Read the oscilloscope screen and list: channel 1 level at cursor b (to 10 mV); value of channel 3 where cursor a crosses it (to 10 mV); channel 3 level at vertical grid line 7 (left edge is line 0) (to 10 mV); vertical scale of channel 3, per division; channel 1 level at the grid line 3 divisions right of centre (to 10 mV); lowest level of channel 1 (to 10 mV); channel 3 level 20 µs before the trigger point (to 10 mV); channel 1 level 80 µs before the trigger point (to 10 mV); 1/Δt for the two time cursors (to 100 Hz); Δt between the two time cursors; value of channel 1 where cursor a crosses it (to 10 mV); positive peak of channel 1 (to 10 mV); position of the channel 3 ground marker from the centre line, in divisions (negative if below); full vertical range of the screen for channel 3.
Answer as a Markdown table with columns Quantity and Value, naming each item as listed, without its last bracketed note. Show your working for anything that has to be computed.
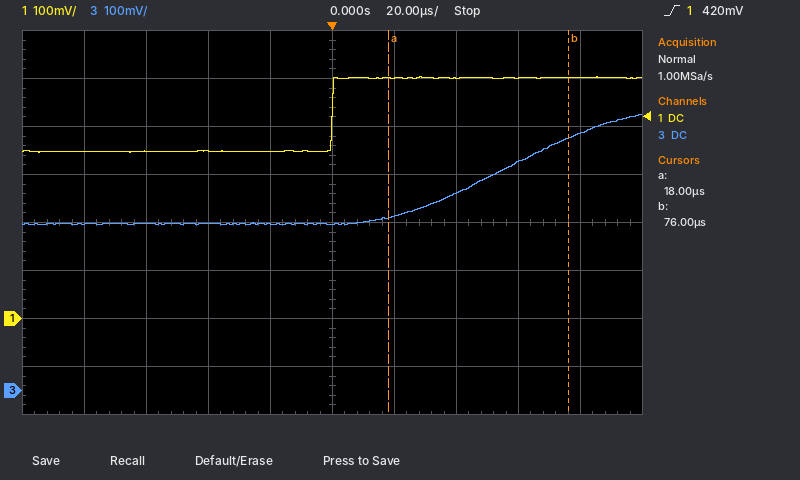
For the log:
| Quantity | Value |
|---|---|
| channel 1 level at cursor b | 500 mV |
| value of channel 3 where cursor a crosses it | 360 mV |
| channel 3 level at vertical grid line 7 (left edge is line 0) | 410 mV |
| vertical scale of channel 3, per division | 100 mV |
| channel 1 level at the grid line 3 divisions right of centre | 500 mV |
| lowest level of channel 1 | 350 mV |
| channel 3 level 20 µs before the trigger point | 350 mV |
| channel 1 level 80 µs before the trigger point | 350 mV |
| 1/Δt for the two time cursors | 1 / 58 µs ≈ 17.2 kHz |
| Δt between the two time cursors | 76 µs − (18 µs) = 58 µs |
| value of channel 1 where cursor a crosses it | 500 mV |
| positive peak of channel 1 | 500 mV |
| position of the channel 3 ground marker from the centre line, in divisions | -3.5 div |
| full vertical range of the screen for channel 3 | 800 mV |
